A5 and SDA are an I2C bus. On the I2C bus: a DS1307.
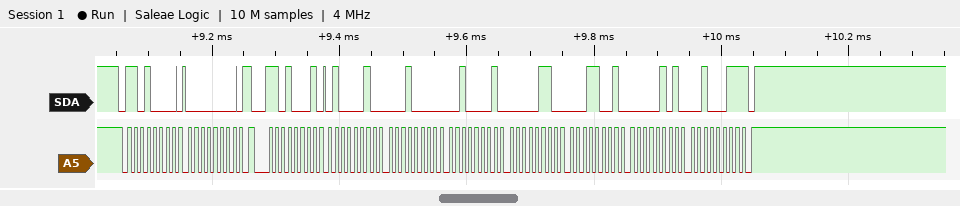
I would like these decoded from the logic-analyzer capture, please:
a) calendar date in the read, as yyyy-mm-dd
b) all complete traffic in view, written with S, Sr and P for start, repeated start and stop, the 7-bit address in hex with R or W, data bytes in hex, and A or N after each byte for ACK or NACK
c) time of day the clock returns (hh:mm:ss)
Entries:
2023-05-19
S 68W A 00 A Sr 68R A 42 A 10 A 21 A 06 A 19 A 05 A 23 N P
21:10:42
